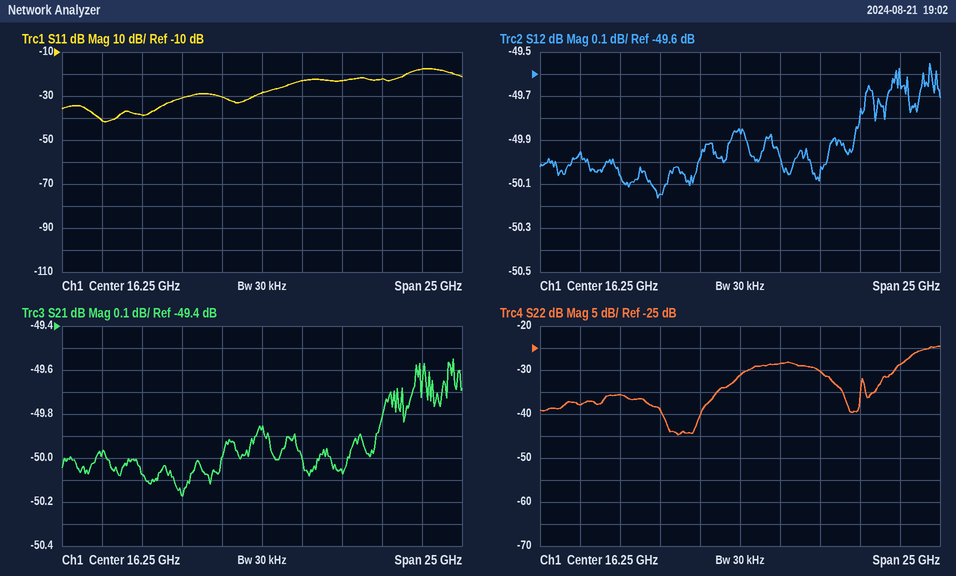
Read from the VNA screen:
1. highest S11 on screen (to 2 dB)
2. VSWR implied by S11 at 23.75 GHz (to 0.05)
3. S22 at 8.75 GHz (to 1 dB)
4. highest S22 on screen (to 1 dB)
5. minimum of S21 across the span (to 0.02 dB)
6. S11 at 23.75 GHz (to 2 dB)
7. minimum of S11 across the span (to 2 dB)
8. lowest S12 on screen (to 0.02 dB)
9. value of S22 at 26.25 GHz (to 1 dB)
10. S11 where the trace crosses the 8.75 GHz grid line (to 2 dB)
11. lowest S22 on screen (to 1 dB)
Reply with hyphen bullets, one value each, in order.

- -18 dB
- 1.15
- -36 dB
- -25 dB
- -50.18 dB
- -22 dB
- -42 dB
- -50.16 dB
- -29 dB
- -38 dB
- -45 dB
